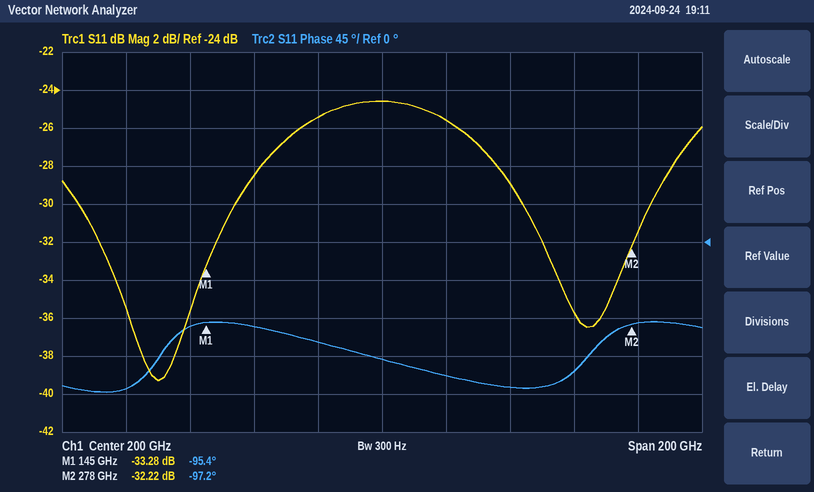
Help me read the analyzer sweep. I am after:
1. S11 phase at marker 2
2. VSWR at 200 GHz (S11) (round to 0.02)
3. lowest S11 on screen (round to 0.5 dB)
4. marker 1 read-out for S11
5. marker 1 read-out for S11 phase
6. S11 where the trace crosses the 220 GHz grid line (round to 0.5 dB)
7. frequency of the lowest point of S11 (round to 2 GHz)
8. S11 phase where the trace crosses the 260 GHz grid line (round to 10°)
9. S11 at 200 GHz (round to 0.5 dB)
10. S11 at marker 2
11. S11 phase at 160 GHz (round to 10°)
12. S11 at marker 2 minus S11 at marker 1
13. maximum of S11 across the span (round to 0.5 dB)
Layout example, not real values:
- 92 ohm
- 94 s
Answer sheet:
- -97.2°
- 1.12
- -39.5 dB
- -33.28 dB
- -95.4°
- -25.5 dB
- 130 GHz
- -150°
- -24.5 dB
- -32.22 dB
- -100°
- 1.06 dB
- -24.5 dB
